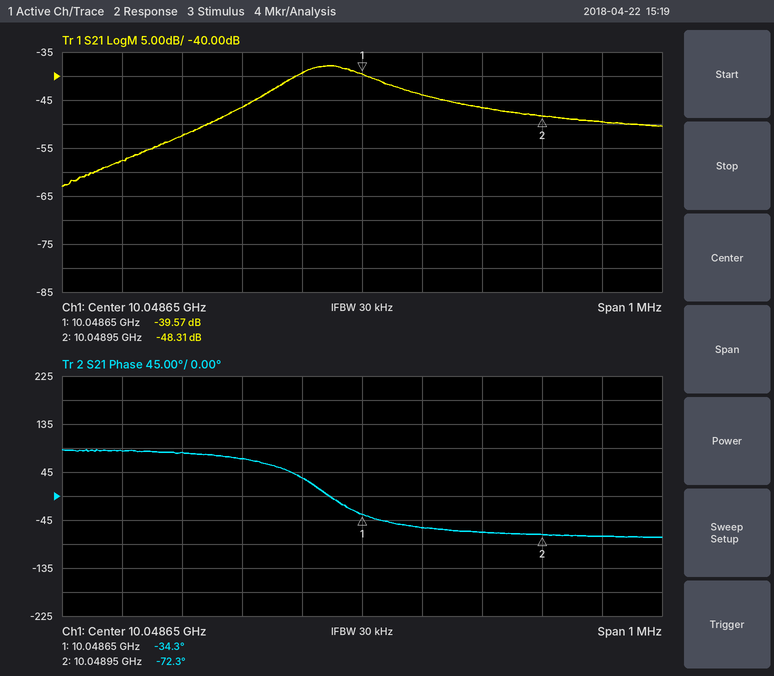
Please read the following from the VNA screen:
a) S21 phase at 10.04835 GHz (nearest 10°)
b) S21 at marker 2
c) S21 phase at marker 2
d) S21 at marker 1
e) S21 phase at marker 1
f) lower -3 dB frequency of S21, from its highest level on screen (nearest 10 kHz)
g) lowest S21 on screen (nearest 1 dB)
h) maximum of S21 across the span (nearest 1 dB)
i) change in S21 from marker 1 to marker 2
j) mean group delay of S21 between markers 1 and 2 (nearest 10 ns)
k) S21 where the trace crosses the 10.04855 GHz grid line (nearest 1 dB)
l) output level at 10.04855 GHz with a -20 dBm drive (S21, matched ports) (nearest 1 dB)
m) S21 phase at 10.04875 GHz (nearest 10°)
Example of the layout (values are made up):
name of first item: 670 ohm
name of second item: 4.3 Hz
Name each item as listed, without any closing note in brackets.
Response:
S21 phase at 10.04835 GHz: 80°
S21 at marker 2: -48.31 dB
S21 phase at marker 2: -72.3°
S21 at marker 1: -39.57 dB
S21 phase at marker 1: -34.3°
lower -3 dB frequency of S21, from its highest level on screen: 10.04853 GHz
lowest S21 on screen: -63 dB
maximum of S21 across the span: -38 dB
change in S21 from marker 1 to marker 2: -8.74 dB
mean group delay of S21 between markers 1 and 2: 350 ns
S21 where the trace crosses the 10.04855 GHz grid line: -39 dB
output level at 10.04855 GHz with a -20 dBm drive (S21, matched ports): -59 dBm
S21 phase at 10.04875 GHz: -60°
